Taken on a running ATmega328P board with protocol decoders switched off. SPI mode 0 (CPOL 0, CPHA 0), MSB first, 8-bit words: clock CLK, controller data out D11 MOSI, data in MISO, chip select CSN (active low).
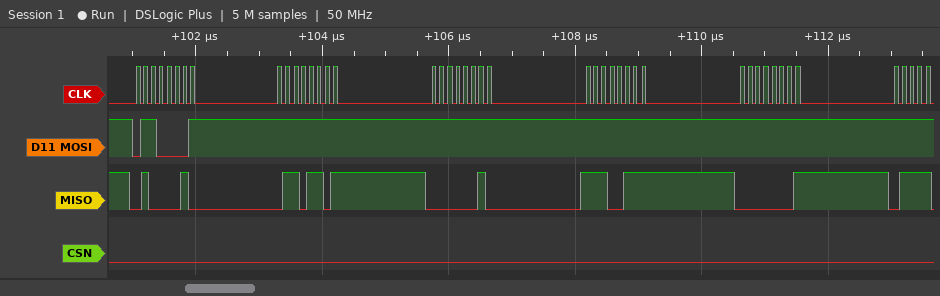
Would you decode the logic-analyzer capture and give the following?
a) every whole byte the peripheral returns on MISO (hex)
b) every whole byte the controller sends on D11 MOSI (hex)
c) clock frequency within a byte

42 6D 02 E7 01
61 FF FF FF FF
8 MHz
